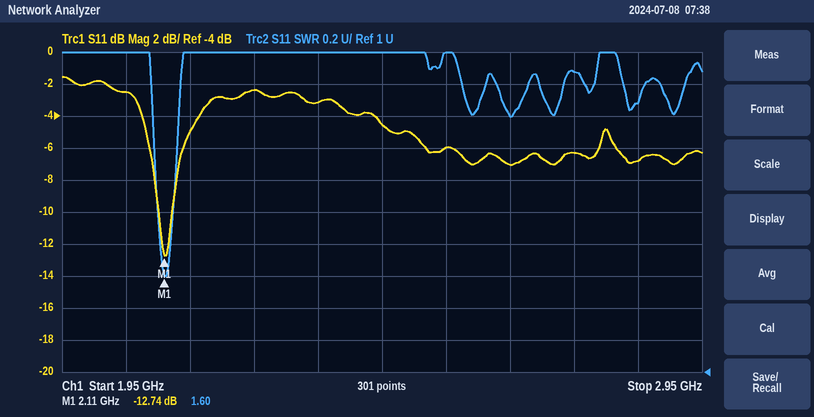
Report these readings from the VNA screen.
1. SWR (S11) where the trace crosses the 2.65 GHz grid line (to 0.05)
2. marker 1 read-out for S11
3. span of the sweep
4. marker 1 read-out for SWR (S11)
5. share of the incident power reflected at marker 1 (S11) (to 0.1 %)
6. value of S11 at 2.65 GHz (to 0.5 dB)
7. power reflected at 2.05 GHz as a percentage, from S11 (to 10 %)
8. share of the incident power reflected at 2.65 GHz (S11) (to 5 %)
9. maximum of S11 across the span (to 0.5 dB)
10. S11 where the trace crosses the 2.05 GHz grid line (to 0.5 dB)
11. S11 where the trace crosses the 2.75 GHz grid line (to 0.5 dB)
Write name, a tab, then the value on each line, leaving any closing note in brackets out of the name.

SWR (S11) where the trace crosses the 2.65 GHz grid line	2.60
marker 1 read-out for S11	-12.74 dB
span of the sweep	1 GHz
marker 1 read-out for SWR	1.60
share of the incident power reflected at marker 1 (S11)	5.3 %
value of S11 at 2.65 GHz	-7.0 dB
power reflected at 2.05 GHz as a percentage, from S11	60 %
share of the incident power reflected at 2.65 GHz (S11)	20 %
maximum of S11 across the span	-1.5 dB
S11 where the trace crosses the 2.05 GHz grid line	-2.5 dB
S11 where the trace crosses the 2.75 GHz grid line	-6.5 dB
